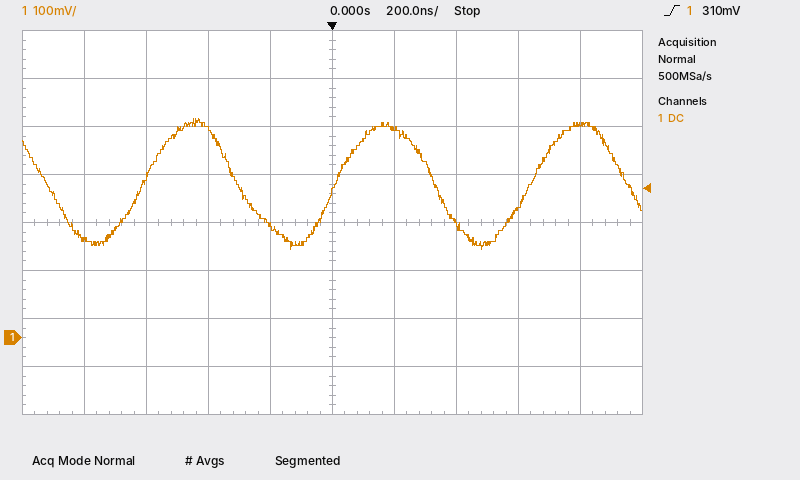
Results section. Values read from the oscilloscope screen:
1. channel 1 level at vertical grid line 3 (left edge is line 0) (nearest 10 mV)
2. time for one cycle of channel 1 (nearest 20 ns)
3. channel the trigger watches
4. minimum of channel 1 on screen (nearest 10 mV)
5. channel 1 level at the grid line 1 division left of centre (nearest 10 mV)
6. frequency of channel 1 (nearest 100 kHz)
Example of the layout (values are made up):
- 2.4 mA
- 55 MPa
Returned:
- 430 mV
- 620 ns
- channel 1
- 180 mV
- 230 mV
- 1.6 MHz
